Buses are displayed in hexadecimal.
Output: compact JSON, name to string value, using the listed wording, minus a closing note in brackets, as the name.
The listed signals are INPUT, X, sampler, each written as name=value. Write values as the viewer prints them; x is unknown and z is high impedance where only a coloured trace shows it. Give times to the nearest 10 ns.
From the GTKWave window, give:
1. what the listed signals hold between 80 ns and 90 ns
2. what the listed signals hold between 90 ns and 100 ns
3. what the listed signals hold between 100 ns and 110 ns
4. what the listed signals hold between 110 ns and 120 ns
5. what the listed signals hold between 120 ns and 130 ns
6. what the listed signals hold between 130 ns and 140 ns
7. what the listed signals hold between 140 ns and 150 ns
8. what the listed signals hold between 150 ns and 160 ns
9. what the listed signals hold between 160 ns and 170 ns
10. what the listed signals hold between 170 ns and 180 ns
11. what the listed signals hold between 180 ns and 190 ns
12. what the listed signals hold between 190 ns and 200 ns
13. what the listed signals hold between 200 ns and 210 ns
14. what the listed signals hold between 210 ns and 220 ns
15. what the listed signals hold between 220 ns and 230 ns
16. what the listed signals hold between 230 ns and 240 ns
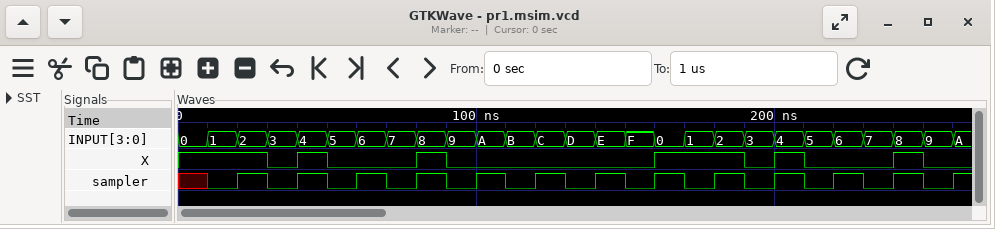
{"what the listed signals hold between 80 ns and 90 ns": "INPUT=8, X=1, sampler=1", "what the listed signals hold between 90 ns and 100 ns": "INPUT=9, X=0, sampler=0", "what the listed signals hold between 100 ns and 110 ns": "INPUT=A, X=0, sampler=1", "what the listed signals hold between 110 ns and 120 ns": "INPUT=B, X=0, sampler=0", "what the listed signals hold between 120 ns and 130 ns": "INPUT=C, X=0, sampler=1", "what the listed signals hold between 130 ns and 140 ns": "INPUT=D, X=0, sampler=0", "what the listed signals hold between 140 ns and 150 ns": "INPUT=E, X=0, sampler=1", "what the listed signals hold between 150 ns and 160 ns": "INPUT=F, X=0, sampler=0", "what the listed signals hold between 160 ns and 170 ns": "INPUT=0, X=1, sampler=1", "what the listed signals hold between 170 ns and 180 ns": "INPUT=1, X=1, sampler=0", "what the listed signals hold between 180 ns and 190 ns": "INPUT=2, X=1, sampler=1", "what the listed signals hold between 190 ns and 200 ns": "INPUT=3, X=0, sampler=0", "what the listed signals hold between 200 ns and 210 ns": "INPUT=4, X=1, sampler=1", "what the listed signals hold between 210 ns and 220 ns": "INPUT=5, X=0, sampler=0", "what the listed signals hold between 220 ns and 230 ns": "INPUT=6, X=0, sampler=1", "what the listed signals hold between 230 ns and 240 ns": "INPUT=7, X=0, sampler=0"}
